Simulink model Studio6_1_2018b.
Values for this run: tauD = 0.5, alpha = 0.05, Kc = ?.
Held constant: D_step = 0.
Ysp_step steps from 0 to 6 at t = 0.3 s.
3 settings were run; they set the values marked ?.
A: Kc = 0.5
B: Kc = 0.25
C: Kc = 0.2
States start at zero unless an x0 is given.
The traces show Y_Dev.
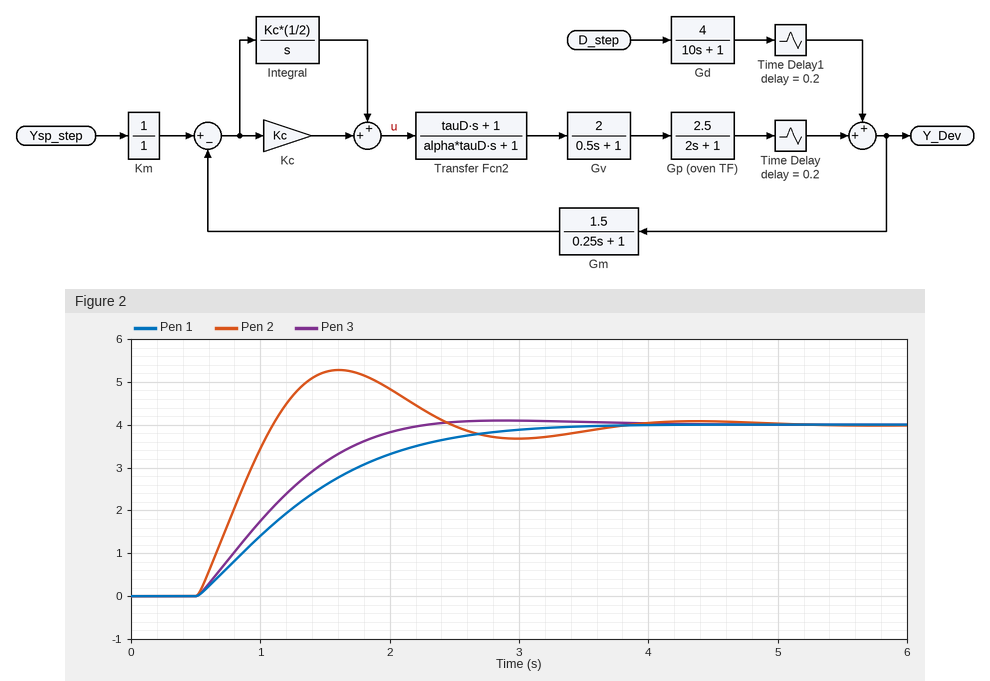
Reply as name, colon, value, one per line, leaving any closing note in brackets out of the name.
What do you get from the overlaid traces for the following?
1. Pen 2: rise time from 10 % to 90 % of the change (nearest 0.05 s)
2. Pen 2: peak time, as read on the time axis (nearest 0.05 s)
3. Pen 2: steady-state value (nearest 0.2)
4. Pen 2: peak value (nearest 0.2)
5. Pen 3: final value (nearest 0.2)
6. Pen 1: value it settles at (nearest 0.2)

Pen 2: rise time from 10 % to 90 % of the change: 0.45 s
Pen 2: peak time, as read on the time axis: 1.60 s
Pen 2: steady-state value: 4.0
Pen 2: peak value: 5.2
Pen 3: final value: 4.0
Pen 1: value it settles at: 4.0
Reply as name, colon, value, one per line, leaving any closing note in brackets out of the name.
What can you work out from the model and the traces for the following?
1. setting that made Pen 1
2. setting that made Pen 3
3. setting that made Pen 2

setting that made Pen 1: C
setting that made Pen 3: B
setting that made Pen 2: A
